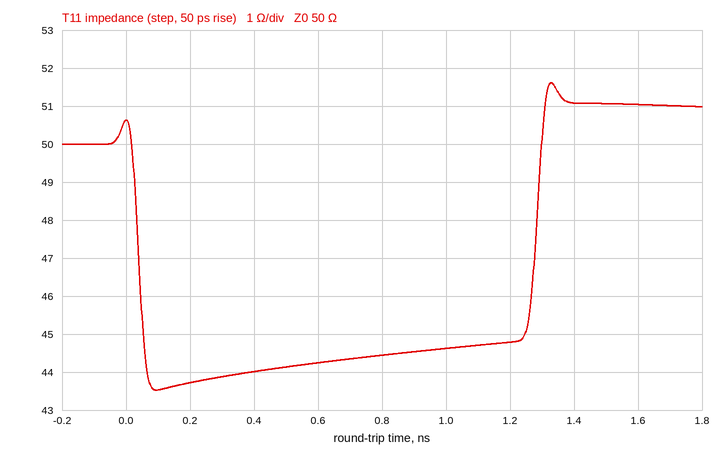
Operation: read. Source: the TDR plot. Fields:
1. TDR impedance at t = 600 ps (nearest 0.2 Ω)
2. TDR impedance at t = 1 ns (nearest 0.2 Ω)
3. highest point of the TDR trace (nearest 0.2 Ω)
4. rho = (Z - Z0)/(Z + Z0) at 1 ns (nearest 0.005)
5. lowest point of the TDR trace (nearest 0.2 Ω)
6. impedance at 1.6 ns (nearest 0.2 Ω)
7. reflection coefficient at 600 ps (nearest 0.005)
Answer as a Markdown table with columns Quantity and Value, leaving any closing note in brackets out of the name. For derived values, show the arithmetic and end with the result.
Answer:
| Quantity | Value |
|---|---|
| TDR impedance at t = 600 ps | 44.2 Ω |
| TDR impedance at t = 1 ns | 44.6 Ω |
| highest point of the TDR trace | 51.6 Ω |
| rho = (Z - Z0)/(Z + Z0) at 1 ns | (44.6 − 50)/(44.6 + 50) ≈ -0.0571, so -0.055 to the nearest 0.005 |
| lowest point of the TDR trace | 43.6 Ω |
| impedance at 1.6 ns | 51.0 Ω |
| reflection coefficient at 600 ps | (44.2 − 50)/(44.2 + 50) ≈ -0.0616, so -0.060 to the nearest 0.005 |
